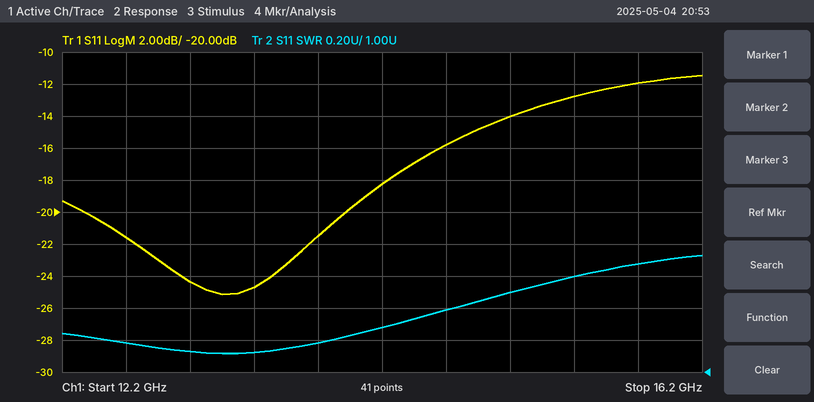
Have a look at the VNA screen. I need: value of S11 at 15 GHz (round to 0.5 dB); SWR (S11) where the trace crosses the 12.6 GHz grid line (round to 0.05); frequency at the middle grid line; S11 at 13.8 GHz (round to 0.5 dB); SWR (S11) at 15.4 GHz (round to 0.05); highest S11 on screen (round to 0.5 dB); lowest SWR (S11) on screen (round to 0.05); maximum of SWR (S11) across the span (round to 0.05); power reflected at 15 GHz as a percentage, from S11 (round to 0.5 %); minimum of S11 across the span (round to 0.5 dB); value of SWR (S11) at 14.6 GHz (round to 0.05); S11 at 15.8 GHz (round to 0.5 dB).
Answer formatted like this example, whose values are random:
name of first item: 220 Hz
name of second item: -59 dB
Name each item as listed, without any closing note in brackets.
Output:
value of S11 at 15 GHz: -14.0 dB
SWR (S11) where the trace crosses the 12.6 GHz grid line: 1.20
frequency at the middle grid line: 14.2 GHz
S11 at 13.8 GHz: -21.5 dB
SWR (S11) at 15.4 GHz: 1.60
highest S11 on screen: -11.5 dB
lowest SWR (S11) on screen: 1.10
maximum of SWR (S11) across the span: 1.75
power reflected at 15 GHz as a percentage, from S11: 4.0 %
minimum of S11 across the span: -25.0 dB
value of SWR (S11) at 14.6 GHz: 1.40
S11 at 15.8 GHz: -12.0 dB
